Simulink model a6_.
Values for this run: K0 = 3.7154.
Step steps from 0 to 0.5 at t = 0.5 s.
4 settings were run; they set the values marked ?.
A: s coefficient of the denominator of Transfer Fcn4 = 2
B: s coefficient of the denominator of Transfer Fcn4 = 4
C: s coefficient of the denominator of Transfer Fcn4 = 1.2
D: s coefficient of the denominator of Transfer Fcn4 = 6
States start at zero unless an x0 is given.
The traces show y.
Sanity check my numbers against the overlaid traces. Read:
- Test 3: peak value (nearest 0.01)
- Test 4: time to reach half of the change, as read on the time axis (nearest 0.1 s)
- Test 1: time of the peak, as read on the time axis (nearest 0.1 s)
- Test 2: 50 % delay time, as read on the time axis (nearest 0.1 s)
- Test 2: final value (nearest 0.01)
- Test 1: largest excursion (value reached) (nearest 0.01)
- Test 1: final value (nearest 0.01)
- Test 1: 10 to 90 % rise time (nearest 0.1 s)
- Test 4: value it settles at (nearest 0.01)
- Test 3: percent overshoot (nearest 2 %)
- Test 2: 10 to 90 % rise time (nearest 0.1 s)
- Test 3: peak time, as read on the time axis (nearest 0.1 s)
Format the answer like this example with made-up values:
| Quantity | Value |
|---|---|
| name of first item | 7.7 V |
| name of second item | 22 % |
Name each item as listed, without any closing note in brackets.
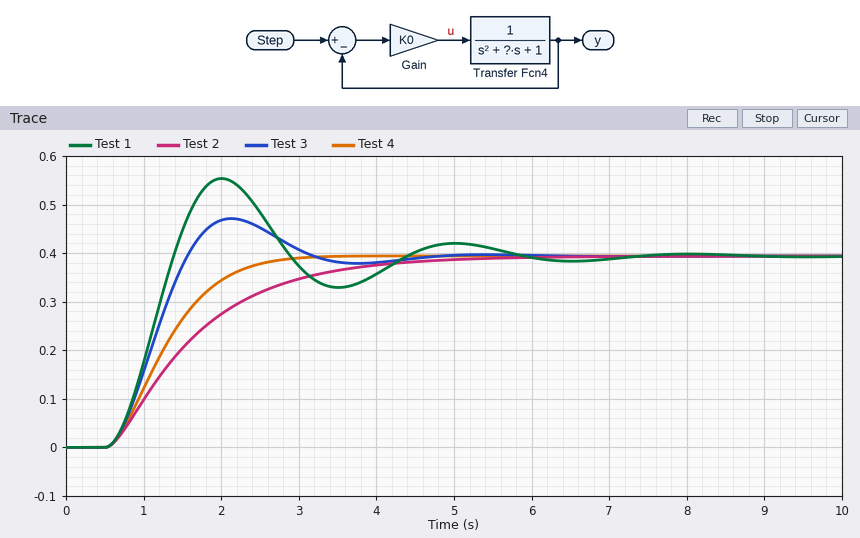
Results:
| Quantity | Value |
|---|---|
| Test 3: peak value | 0.47 |
| Test 4: time to reach half of the change, as read on the time axis | 1.2 s |
| Test 1: time of the peak, as read on the time axis | 2.0 s |
| Test 2: 50 % delay time, as read on the time axis | 1.5 s |
| Test 2: final value | 0.39 |
| Test 1: largest excursion (value reached) | 0.55 |
| Test 1: final value | 0.39 |
| Test 1: 10 to 90 % rise time | 0.6 s |
| Test 4: value it settles at | 0.39 |
| Test 3: percent overshoot | 20 % |
| Test 2: 10 to 90 % rise time | 2.4 s |
| Test 3: peak time, as read on the time axis | 2.1 s |
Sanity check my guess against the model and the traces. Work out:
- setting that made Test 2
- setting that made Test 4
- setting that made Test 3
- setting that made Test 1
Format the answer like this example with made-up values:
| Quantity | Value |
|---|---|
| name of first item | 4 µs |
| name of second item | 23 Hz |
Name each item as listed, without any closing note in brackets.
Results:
| Quantity | Value |
|---|---|
| setting that made Test 2 | D |
| setting that made Test 4 | B |
| setting that made Test 3 | A |
| setting that made Test 1 | C |
